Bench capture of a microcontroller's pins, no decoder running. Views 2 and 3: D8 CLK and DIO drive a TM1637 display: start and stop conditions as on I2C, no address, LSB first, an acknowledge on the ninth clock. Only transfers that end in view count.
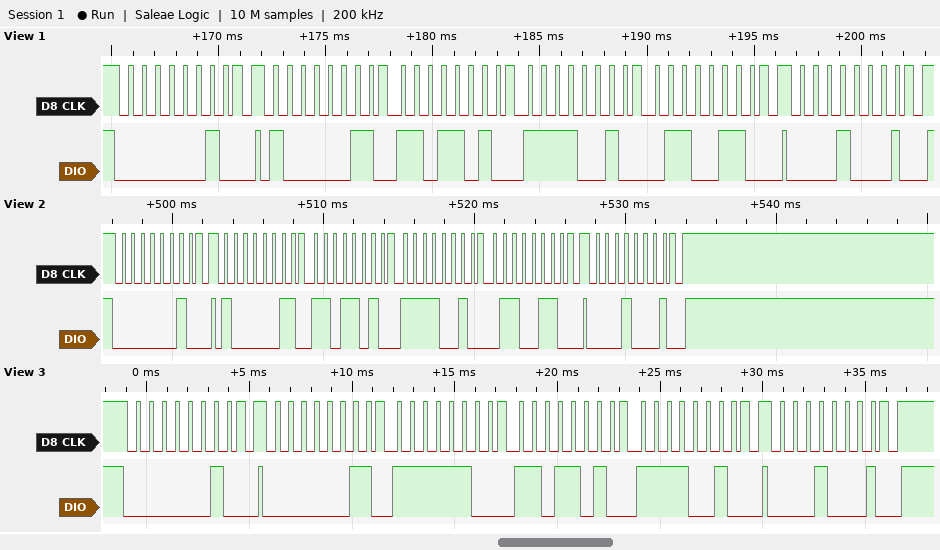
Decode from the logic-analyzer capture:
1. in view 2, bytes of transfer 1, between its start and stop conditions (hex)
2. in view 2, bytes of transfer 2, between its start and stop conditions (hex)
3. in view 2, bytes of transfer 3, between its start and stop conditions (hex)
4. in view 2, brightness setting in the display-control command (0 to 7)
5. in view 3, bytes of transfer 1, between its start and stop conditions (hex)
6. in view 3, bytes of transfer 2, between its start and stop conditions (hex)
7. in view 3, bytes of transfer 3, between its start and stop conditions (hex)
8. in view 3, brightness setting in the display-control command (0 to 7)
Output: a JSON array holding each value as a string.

["40", "C1 5B 4F 66", "88", "0", "40", "C0 3F 5B 4F", "88", "0"]
